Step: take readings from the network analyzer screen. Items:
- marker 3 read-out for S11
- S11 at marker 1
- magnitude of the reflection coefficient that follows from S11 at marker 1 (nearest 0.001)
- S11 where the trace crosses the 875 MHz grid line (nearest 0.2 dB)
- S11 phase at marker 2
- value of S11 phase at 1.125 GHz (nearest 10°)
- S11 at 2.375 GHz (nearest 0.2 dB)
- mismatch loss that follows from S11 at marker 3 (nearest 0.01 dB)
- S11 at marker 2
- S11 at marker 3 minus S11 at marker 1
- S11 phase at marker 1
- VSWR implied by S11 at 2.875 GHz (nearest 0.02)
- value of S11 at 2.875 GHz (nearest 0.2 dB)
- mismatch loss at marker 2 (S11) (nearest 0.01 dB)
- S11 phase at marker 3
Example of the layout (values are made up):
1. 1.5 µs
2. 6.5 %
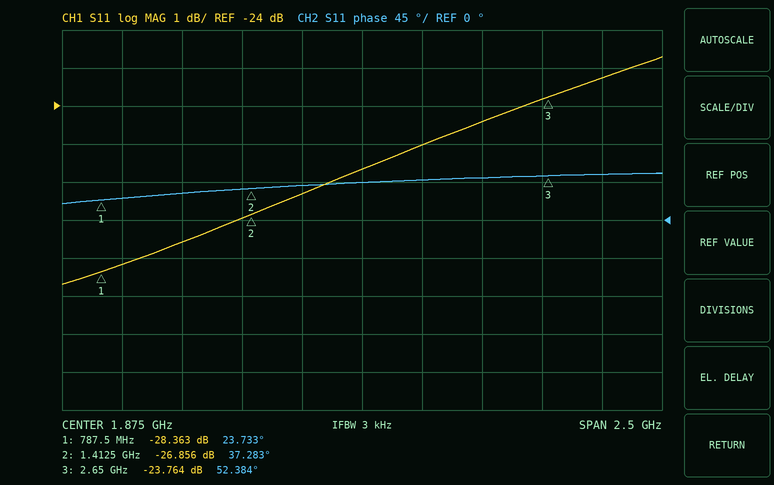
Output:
1. -23.764 dB
2. -28.363 dB
3. 0.038
4. -28.2 dB
5. 37.283°
6. 30°
7. -24.4 dB
8. 0.02 dB
9. -26.856 dB
10. 4.599 dB
11. 23.733°
12. 1.14
13. -23.2 dB
14. 0.01 dB
15. 52.384°
